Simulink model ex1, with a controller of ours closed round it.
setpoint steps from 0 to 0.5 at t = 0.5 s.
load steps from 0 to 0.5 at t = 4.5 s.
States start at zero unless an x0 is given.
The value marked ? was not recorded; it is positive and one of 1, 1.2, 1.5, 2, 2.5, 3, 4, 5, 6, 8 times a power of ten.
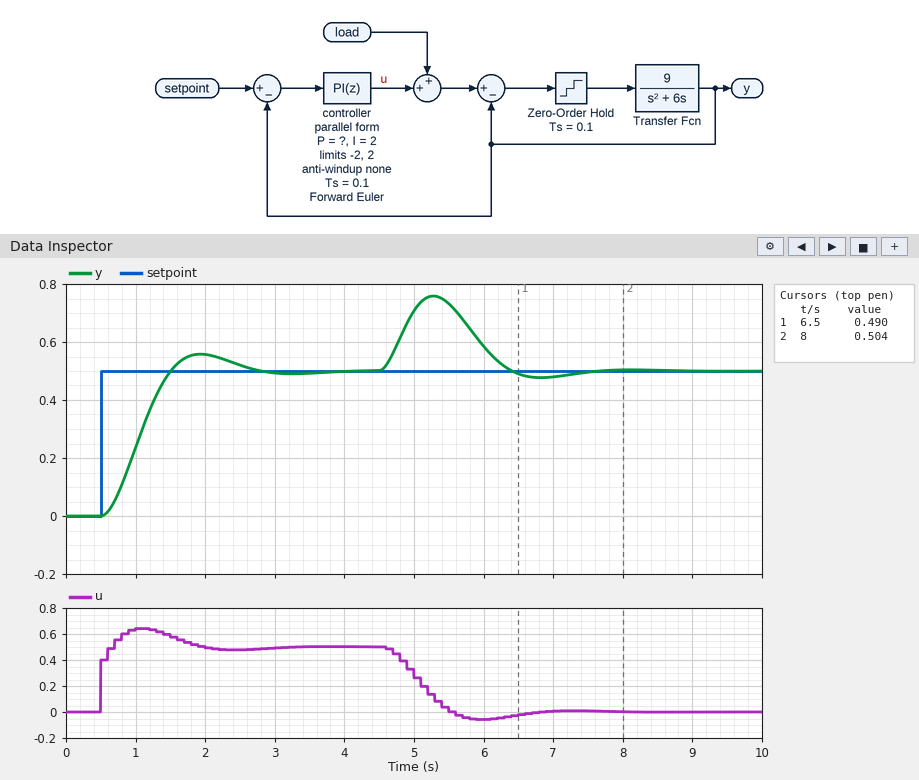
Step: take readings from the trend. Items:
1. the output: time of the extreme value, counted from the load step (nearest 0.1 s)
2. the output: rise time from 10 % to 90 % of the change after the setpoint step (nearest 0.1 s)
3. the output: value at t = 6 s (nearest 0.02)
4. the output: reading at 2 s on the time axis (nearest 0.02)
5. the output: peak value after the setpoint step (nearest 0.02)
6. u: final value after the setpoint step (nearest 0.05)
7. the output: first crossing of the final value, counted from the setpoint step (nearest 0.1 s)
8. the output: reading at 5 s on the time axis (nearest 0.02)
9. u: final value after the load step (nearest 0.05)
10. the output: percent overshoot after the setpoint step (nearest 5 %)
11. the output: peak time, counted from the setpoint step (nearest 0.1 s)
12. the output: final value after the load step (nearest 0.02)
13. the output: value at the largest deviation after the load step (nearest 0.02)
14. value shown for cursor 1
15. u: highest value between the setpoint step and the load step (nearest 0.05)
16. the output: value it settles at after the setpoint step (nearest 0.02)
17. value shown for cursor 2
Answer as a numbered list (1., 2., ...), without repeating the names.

1. 0.8 s
2. 0.7 s
3. 0.58
4. 0.56
5. 0.56
6. 0.50
7. 1.0 s
8. 0.70
9. 0.00
10. 10 %
11. 1.4 s
12. 0.50
13. 0.76
14. 0.490
15. 0.65
16. 0.50
17. 0.504
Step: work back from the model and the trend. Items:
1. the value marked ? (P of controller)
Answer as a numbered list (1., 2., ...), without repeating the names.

1. 0.8
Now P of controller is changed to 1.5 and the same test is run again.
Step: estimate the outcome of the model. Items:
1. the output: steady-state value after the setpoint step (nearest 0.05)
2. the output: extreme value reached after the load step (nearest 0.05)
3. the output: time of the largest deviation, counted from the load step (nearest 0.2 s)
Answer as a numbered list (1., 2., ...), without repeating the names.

1. 0.50
2. 0.70
3. 0.6 s
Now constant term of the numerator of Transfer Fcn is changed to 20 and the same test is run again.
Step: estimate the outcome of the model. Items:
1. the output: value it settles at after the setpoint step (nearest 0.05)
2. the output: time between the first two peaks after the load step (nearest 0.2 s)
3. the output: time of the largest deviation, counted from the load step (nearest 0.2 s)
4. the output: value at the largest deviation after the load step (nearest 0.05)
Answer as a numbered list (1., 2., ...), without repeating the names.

1. 0.50
2. 1.2 s
3. 0.6 s
4. 0.85
